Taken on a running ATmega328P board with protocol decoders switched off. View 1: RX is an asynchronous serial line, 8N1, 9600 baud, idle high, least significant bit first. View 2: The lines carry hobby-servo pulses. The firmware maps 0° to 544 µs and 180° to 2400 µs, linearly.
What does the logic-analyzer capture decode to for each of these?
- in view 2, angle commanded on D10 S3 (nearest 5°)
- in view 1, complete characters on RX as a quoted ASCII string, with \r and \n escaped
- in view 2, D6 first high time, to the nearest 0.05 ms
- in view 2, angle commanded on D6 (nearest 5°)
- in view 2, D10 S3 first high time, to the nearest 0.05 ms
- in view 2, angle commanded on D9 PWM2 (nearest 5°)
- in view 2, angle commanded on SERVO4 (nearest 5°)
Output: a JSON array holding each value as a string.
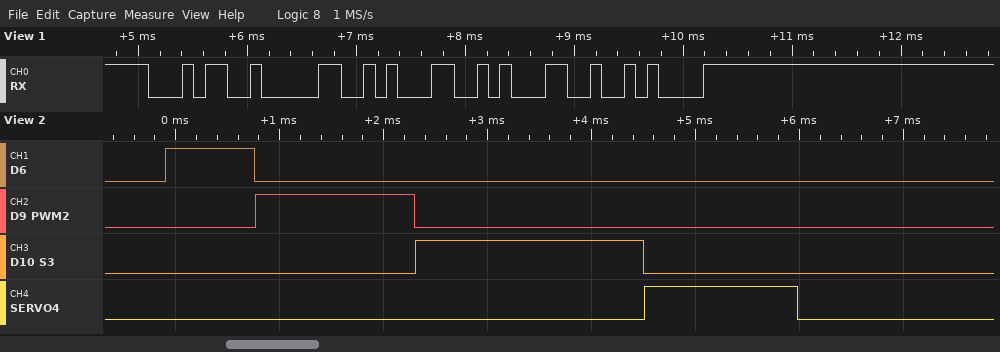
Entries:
["160°", "\"4011\\n\"", "0.85 ms", "30°", "2.20 ms", "95°", "90°"]
